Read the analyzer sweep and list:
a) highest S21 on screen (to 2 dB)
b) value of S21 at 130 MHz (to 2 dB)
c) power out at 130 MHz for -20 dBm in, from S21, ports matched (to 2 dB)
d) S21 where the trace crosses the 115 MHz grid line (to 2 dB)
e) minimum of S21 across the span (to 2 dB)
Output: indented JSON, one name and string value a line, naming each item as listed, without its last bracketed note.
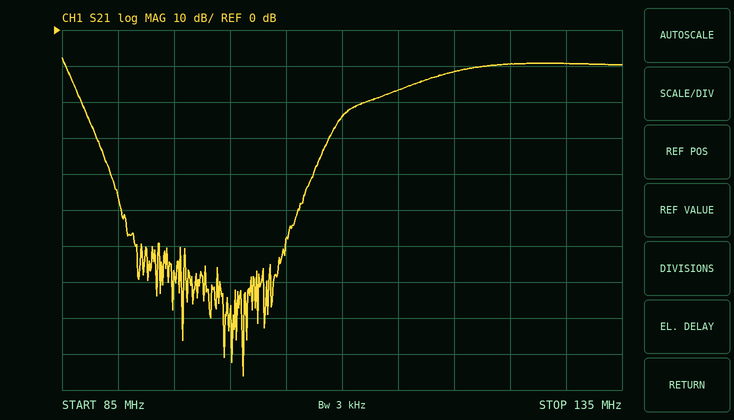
{
  "highest S21 on screen": "-8 dB",
  "value of S21 at 130 MHz": "-10 dB",
  "power out at 130 MHz for -20 dBm in, from S21, ports matched": "-30 dBm",
  "S21 where the trace crosses the 115 MHz grid line": "-16 dB",
  "minimum of S21 across the span": "-96 dB"
}
